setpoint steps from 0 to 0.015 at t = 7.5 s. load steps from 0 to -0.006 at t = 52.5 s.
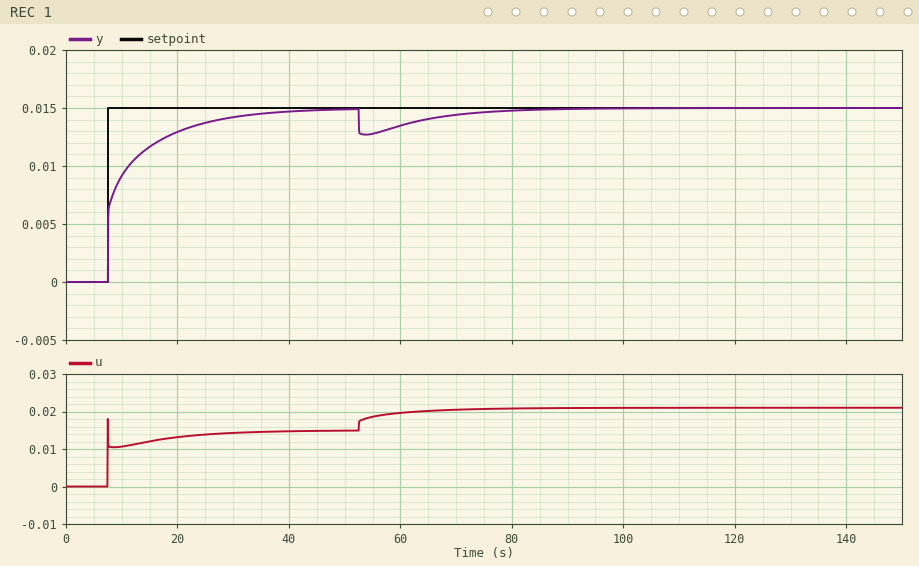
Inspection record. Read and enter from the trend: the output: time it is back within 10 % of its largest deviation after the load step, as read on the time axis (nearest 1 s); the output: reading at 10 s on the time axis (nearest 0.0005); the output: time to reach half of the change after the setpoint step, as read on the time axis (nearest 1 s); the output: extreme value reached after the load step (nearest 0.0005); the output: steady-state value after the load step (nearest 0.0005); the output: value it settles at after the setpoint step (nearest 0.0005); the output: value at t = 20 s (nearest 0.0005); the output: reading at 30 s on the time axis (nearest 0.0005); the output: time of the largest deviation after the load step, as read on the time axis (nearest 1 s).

80 s
0.0090
8 s
0.0125
0.0150
0.0150
0.0130
0.0140
54 s
